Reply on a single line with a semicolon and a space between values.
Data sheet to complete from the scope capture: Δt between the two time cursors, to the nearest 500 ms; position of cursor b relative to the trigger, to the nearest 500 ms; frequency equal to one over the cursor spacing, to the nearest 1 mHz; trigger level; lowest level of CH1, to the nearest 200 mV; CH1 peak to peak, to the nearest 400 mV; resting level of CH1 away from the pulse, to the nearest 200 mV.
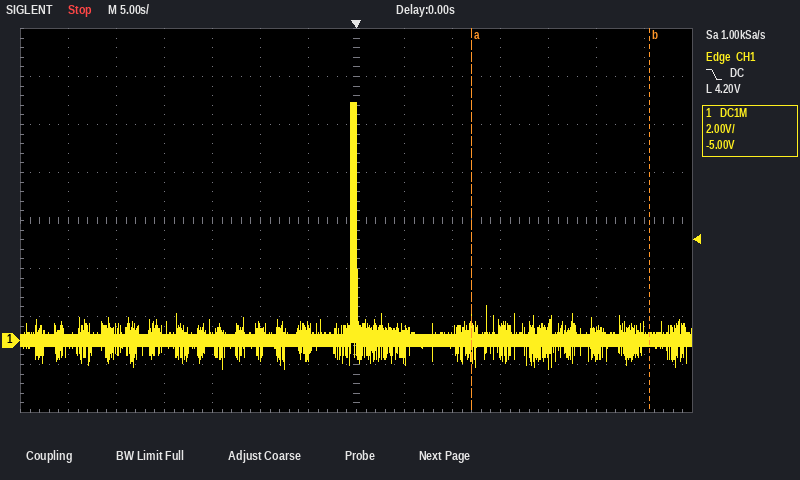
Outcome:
18.5 s; +30.5 s; 54 mHz; 4.20 V; -1.2 V; 11.2 V; 0.0 V
